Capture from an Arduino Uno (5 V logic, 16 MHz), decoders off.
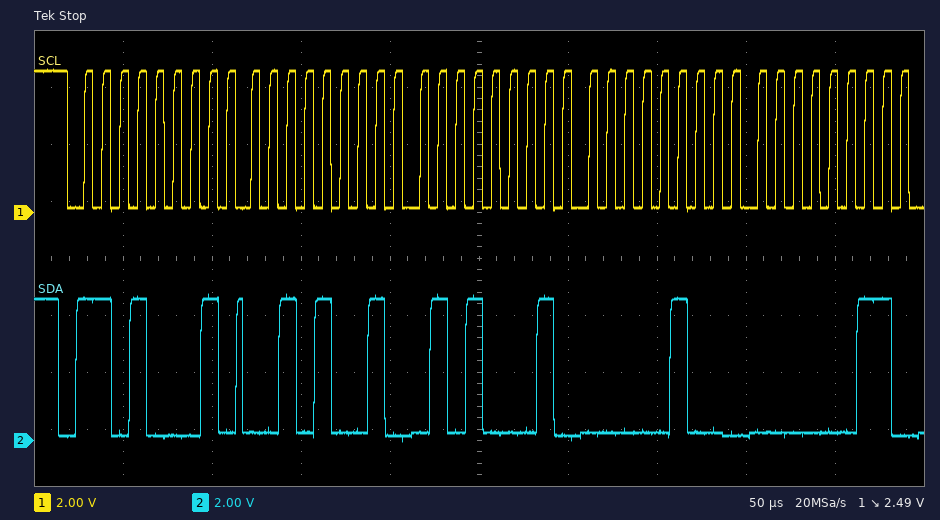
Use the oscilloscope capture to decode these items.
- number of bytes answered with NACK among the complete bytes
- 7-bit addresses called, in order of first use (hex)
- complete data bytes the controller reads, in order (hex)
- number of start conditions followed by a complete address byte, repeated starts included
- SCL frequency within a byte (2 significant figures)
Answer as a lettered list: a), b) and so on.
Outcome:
a) 0
b) 0x68
c) 29 51 04 03
d) 1
e) 100 kHz
